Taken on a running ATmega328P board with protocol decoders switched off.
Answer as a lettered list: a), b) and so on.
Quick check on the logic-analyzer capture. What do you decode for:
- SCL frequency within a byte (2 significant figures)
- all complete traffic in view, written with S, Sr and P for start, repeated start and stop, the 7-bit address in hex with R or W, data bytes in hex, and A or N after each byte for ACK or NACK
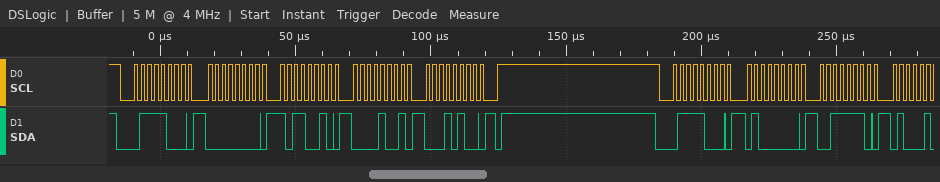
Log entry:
a) 400 kHz
b) S 3CW A 00 A B2 A 09 A 14 A P S 3CW A 40 A 3E A
